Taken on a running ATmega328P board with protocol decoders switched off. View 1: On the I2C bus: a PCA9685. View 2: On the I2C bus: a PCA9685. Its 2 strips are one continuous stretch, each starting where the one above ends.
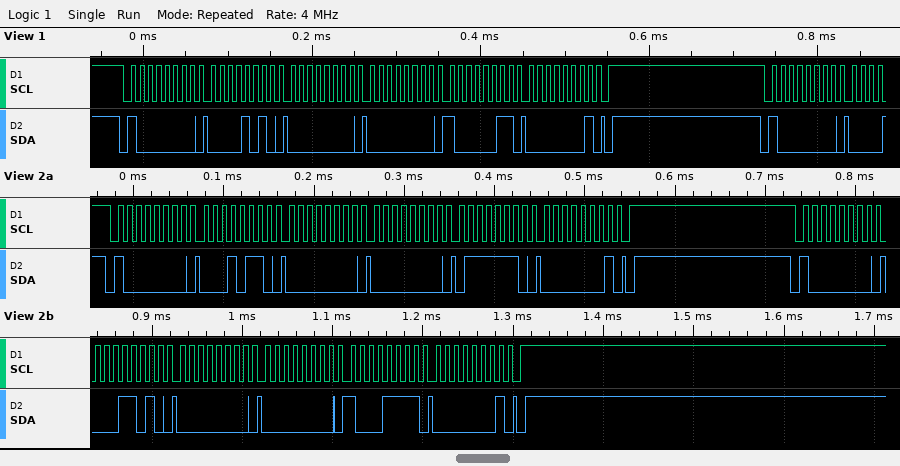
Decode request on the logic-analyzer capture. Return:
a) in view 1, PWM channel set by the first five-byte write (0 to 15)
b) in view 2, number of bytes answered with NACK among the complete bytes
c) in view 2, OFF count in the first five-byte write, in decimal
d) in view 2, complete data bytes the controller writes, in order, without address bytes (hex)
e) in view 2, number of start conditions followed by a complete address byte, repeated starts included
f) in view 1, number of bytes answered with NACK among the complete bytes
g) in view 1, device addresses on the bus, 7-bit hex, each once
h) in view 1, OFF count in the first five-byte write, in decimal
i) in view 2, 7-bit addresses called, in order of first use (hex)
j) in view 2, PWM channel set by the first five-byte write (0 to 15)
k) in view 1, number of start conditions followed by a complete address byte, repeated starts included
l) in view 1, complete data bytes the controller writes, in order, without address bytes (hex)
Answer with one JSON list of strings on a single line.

["1", "0", "382", "16 00 00 7E 01 1A 00 00 8F 01", "2", "0", "0x40", "387", "0x40", "4", "2", "0A 00 00 83 01"]
